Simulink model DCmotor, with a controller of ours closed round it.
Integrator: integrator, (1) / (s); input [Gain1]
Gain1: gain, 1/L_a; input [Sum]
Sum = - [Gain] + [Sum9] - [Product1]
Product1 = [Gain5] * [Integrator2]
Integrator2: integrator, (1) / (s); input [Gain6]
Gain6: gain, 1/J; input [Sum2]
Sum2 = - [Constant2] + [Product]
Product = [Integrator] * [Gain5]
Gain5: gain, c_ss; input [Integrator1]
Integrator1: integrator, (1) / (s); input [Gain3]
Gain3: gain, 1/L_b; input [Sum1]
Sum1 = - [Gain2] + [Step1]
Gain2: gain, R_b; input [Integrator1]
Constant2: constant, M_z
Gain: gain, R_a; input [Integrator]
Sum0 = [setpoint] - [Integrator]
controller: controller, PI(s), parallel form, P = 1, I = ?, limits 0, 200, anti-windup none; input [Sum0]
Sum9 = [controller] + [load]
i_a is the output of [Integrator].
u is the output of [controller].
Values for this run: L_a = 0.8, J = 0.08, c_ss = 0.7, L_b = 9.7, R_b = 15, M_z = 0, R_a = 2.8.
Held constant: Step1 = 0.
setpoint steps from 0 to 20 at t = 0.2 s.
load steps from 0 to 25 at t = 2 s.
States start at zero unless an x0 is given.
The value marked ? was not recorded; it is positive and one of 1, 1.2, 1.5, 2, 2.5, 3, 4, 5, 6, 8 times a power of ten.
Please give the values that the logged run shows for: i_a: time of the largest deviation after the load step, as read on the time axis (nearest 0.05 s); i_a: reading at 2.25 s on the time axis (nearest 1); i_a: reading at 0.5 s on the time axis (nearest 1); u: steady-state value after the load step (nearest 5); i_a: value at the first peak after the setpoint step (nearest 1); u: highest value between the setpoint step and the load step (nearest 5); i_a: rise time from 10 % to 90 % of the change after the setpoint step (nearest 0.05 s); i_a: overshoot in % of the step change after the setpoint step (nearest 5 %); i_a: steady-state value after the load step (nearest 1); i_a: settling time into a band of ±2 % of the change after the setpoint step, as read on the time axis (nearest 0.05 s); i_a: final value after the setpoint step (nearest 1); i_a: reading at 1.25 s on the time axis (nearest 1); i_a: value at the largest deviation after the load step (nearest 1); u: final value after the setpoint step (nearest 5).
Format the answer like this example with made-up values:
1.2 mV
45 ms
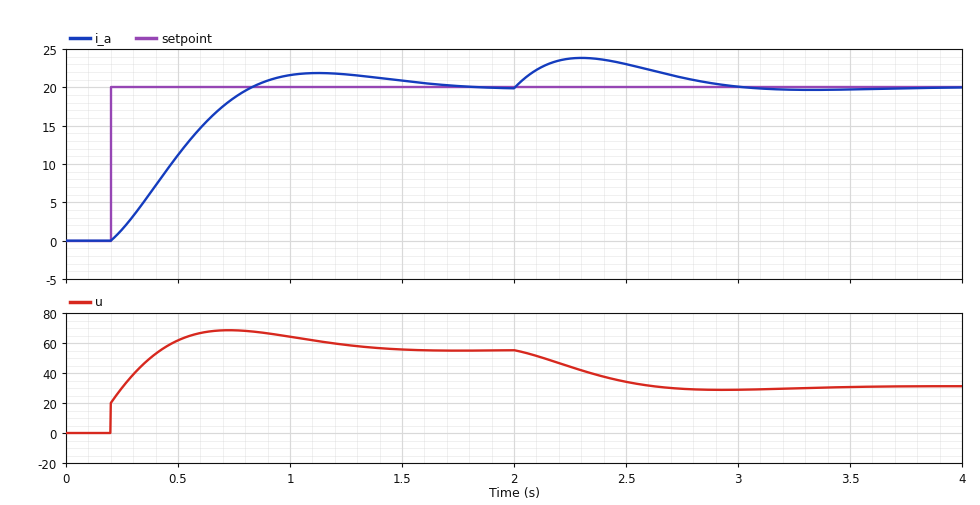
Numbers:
2.30 s
24
11
30
22
70
0.45 s
10 %
20
1.65 s
20
22
24
55
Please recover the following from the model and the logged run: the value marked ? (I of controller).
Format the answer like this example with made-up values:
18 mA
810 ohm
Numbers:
12
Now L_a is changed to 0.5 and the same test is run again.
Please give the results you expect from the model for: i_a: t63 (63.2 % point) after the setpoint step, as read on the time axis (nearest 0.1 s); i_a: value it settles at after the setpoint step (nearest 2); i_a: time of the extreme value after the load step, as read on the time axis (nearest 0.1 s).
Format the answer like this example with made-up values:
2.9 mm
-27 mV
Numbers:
0.5 s
20
2.2 s
